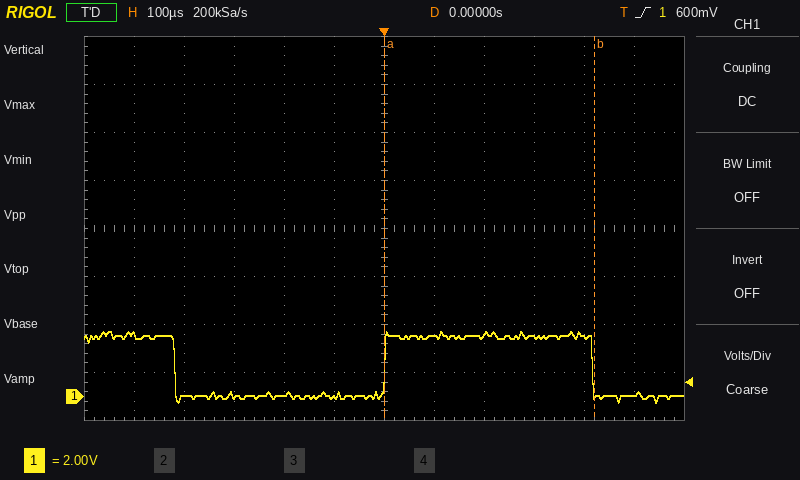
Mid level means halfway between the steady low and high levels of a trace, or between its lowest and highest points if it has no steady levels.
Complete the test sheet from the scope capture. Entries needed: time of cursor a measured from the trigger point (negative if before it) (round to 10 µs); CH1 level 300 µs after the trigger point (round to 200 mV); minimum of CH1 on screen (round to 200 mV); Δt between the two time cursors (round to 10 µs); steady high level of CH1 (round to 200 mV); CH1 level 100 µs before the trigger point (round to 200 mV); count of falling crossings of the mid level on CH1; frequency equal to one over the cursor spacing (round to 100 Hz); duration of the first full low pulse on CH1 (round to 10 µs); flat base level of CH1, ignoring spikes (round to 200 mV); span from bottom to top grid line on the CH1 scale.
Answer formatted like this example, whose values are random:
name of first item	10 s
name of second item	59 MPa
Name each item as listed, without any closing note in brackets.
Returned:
time of cursor a measured from the trigger point (negative if before it)	0 µs
CH1 level 300 µs after the trigger point	2.4 V
minimum of CH1 on screen	-200 mV
Δt between the two time cursors	420 µs
steady high level of CH1	2.6 V
CH1 level 100 µs before the trigger point	0.0 V
count of falling crossings of the mid level on CH1	2
frequency equal to one over the cursor spacing	2.4 kHz
duration of the first full low pulse on CH1	420 µs
flat base level of CH1, ignoring spikes	0.0 V
span from bottom to top grid line on the CH1 scale	16 V
